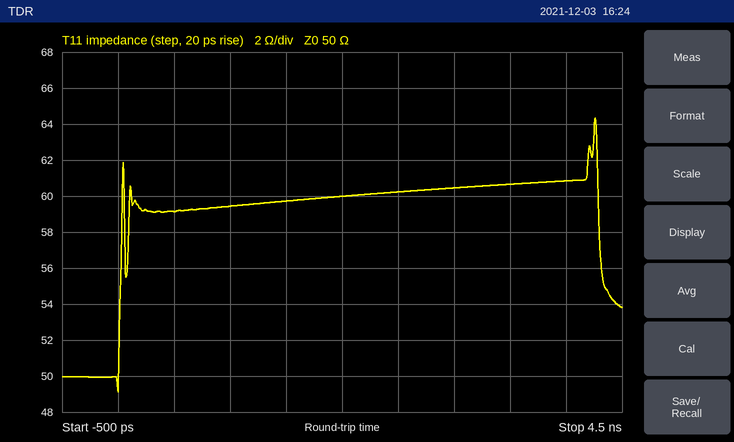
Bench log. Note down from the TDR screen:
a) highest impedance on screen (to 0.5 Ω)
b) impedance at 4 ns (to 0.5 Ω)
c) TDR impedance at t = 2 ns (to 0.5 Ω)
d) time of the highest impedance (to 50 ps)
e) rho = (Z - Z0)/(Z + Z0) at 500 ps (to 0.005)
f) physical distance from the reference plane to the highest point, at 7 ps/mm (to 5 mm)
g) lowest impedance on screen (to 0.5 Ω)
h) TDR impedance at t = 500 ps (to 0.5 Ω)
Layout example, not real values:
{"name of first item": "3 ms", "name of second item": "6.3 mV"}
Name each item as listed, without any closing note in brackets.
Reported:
{"highest impedance on screen": "64.5 Ω", "impedance at 4 ns": "61.0 Ω", "TDR impedance at t = 2 ns": "60.0 Ω", "time of the highest impedance": "4.25 ns", "rho = (Z - Z0)/(Z + Z0) at 500 ps": "+0.085", "physical distance from the reference plane to the highest point, at 7 ps/mm": "305 mm", "lowest impedance on screen": "49.0 Ω", "TDR impedance at t = 500 ps": "59.0 Ω"}
